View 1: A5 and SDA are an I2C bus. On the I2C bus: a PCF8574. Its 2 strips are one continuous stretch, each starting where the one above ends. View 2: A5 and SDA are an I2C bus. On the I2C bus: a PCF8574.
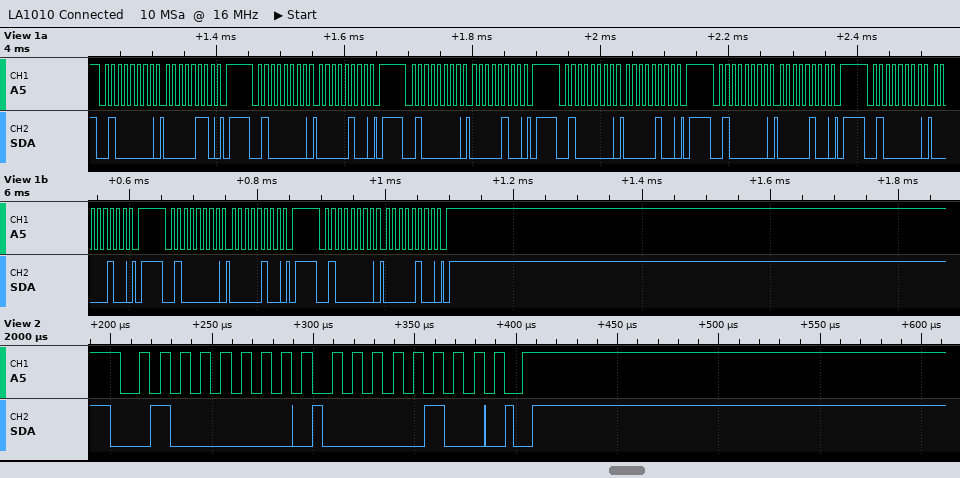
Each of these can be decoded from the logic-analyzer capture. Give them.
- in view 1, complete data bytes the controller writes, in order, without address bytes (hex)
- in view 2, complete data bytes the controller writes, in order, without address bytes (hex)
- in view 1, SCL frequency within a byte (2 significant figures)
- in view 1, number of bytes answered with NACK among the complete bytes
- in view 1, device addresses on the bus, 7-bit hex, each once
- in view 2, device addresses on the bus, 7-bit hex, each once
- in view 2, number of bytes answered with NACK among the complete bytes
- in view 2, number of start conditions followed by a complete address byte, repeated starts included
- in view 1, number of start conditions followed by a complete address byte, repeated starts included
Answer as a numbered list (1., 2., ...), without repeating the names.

1. 06 04 04 04 04 04 04 04
2. 04
3. 100 kHz
4. 0
5. 0x20
6. 0x20
7. 0
8. 1
9. 8
